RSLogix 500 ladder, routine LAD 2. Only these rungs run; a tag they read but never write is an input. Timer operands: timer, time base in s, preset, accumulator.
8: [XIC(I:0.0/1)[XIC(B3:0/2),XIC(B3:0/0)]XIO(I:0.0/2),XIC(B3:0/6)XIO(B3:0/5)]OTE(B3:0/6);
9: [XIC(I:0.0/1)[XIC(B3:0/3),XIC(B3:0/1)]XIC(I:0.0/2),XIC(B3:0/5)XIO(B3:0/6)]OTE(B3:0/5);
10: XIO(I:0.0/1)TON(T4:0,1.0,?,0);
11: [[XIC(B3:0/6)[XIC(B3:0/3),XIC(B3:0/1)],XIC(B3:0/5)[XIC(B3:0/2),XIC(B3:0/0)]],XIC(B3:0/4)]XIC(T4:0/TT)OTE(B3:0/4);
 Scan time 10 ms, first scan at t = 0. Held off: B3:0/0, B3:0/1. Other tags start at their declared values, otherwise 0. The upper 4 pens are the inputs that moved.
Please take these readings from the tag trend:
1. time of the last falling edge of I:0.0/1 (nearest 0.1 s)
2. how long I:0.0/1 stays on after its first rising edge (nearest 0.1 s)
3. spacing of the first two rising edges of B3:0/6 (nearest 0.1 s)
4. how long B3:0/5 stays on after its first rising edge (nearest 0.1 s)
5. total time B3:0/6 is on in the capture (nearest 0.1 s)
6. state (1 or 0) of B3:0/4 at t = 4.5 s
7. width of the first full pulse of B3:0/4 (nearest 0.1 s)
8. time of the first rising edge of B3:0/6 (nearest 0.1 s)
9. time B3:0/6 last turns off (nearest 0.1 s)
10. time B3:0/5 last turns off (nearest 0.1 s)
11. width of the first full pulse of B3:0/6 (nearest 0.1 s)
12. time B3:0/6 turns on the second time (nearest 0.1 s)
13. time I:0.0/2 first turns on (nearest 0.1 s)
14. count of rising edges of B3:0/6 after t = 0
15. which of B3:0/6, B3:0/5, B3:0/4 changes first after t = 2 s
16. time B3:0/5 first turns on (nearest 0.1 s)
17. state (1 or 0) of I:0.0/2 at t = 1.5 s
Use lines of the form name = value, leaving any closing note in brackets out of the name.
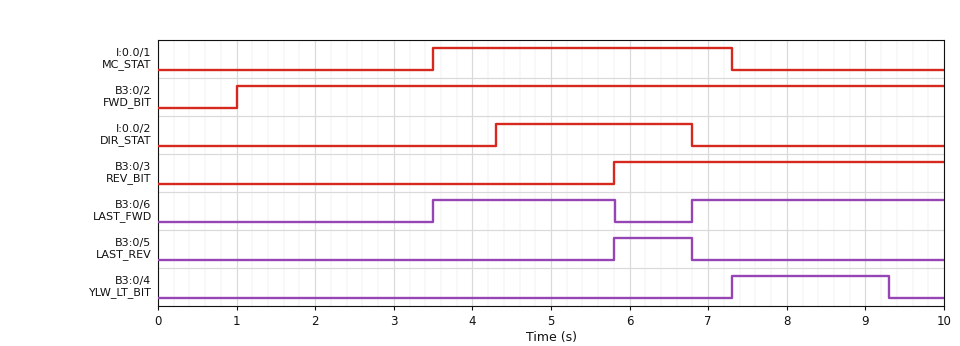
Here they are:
time of the last falling edge of I:0.0/1 = 7.3 s
how long I:0.0/1 stays on after its first rising edge = 3.8 s
spacing of the first two rising edges of B3:0/6 = 3.3 s
how long B3:0/5 stays on after its first rising edge = 1.0 s
total time B3:0/6 is on in the capture = 5.5 s
state (1 or 0) of B3:0/4 at t = 4.5 s = 0
width of the first full pulse of B3:0/4 = 2.0 s
time of the first rising edge of B3:0/6 = 3.5 s
time B3:0/6 last turns off = 5.8 s
time B3:0/5 last turns off = 6.8 s
width of the first full pulse of B3:0/6 = 2.3 s
time B3:0/6 turns on the second time = 6.8 s
time I:0.0/2 first turns on = 4.3 s
count of rising edges of B3:0/6 after t = 0 = 2
which of B3:0/6, B3:0/5, B3:0/4 changes first after t = 2 s = B3:0/6
time B3:0/5 first turns on = 5.8 s
state (1 or 0) of I:0.0/2 at t = 1.5 s = 0
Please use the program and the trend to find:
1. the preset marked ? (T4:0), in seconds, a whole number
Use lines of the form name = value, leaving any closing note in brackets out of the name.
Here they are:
the preset marked ? (T4:0), in seconds, a whole number = 2 s
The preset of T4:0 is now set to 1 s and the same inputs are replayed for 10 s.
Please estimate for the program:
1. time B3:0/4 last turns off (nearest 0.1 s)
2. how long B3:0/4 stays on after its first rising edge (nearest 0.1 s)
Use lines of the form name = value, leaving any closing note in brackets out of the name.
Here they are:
time B3:0/4 last turns off = 8.3 s
how long B3:0/4 stays on after its first rising edge = 1.0 s
